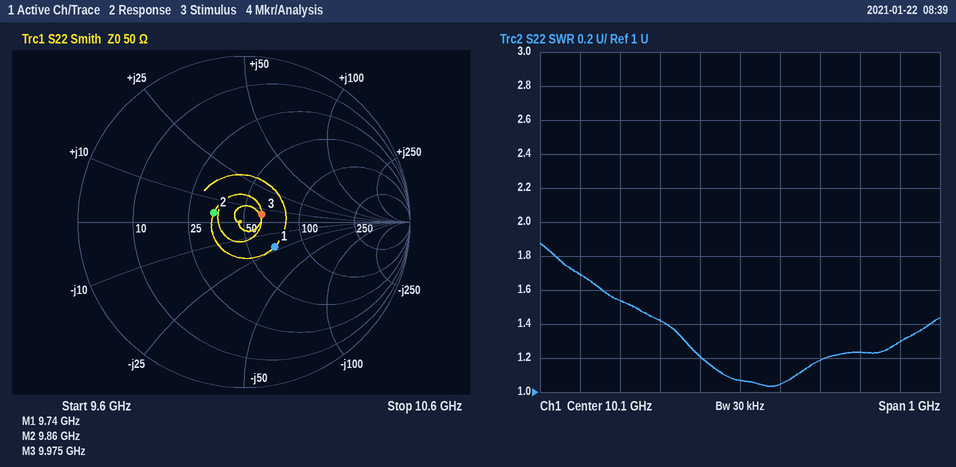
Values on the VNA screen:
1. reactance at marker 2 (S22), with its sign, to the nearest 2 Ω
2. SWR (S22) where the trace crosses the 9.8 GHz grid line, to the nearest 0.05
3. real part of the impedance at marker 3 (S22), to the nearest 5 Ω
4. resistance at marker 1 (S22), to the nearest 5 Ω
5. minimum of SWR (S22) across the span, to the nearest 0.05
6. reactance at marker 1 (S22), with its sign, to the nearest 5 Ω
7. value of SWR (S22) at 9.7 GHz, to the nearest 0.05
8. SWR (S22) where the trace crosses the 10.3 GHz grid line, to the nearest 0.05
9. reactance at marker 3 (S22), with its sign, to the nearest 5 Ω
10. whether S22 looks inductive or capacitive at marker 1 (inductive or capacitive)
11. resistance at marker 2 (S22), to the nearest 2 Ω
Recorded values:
+4 Ω
1.55
60 Ω
70 Ω
1.05
-20 Ω
1.70
1.20
+5 Ω
capacitive
34 Ω
